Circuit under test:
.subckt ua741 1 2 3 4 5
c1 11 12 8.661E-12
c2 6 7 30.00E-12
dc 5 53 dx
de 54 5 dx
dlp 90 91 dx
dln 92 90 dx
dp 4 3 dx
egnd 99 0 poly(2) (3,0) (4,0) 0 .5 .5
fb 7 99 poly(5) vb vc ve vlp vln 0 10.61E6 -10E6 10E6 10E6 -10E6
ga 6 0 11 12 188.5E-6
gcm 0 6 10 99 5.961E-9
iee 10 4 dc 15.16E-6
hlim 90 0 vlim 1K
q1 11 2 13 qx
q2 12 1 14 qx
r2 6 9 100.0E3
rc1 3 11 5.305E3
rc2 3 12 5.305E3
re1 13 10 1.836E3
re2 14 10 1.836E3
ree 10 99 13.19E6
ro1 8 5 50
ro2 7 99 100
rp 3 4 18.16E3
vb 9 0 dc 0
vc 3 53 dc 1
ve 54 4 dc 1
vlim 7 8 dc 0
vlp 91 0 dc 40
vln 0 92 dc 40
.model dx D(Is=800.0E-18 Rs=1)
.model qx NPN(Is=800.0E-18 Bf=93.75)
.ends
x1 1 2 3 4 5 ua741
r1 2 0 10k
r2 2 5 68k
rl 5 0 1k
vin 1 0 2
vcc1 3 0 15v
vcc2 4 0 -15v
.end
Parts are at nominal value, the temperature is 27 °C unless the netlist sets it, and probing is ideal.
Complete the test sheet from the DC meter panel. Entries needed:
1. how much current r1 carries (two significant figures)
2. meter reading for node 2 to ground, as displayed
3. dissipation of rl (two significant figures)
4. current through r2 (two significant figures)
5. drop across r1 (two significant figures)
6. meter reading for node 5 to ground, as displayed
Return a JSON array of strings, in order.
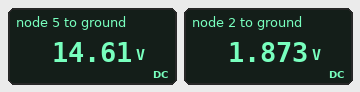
["190 µA", "1.873 V", "210 mW", "190 µA", "1.9 V", "14.61 V"]
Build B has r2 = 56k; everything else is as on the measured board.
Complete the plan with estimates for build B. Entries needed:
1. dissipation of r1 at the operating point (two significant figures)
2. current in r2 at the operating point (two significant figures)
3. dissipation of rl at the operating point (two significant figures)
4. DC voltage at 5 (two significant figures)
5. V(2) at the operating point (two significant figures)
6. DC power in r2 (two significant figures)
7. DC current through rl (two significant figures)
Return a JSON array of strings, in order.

["400 µW", "200 µA", "170 mW", "13 V", "2.0 V", "2.2 mW", "13 mA"]
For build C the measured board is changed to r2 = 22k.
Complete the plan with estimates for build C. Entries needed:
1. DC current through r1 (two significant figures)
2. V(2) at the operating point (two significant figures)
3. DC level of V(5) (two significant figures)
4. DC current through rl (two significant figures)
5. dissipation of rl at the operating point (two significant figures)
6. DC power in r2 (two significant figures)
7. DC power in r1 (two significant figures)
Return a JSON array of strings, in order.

["200 µA", "2.0 V", "6.4 V", "6.4 mA", "41 mW", "880 µW", "400 µW"]
